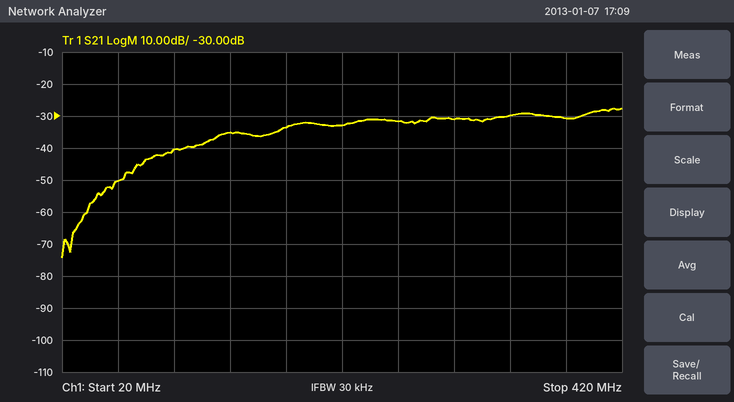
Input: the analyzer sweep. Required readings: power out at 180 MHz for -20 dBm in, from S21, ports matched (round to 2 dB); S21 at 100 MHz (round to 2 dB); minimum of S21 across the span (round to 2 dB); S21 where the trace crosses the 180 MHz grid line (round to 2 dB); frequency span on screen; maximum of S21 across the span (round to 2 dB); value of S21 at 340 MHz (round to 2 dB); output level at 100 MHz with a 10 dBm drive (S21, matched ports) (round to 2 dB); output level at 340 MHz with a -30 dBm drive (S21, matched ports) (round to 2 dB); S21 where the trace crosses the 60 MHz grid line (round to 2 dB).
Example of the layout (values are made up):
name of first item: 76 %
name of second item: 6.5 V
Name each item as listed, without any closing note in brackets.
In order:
power out at 180 MHz for -20 dBm in, from S21, ports matched: -54 dBm
S21 at 100 MHz: -40 dB
minimum of S21 across the span: -74 dB
S21 where the trace crosses the 180 MHz grid line: -34 dB
frequency span on screen: 400 MHz
maximum of S21 across the span: -28 dB
value of S21 at 340 MHz: -30 dB
output level at 100 MHz with a 10 dBm drive (S21, matched ports): -30 dBm
output level at 340 MHz with a -30 dBm drive (S21, matched ports): -60 dBm
S21 where the trace crosses the 60 MHz grid line: -50 dB
